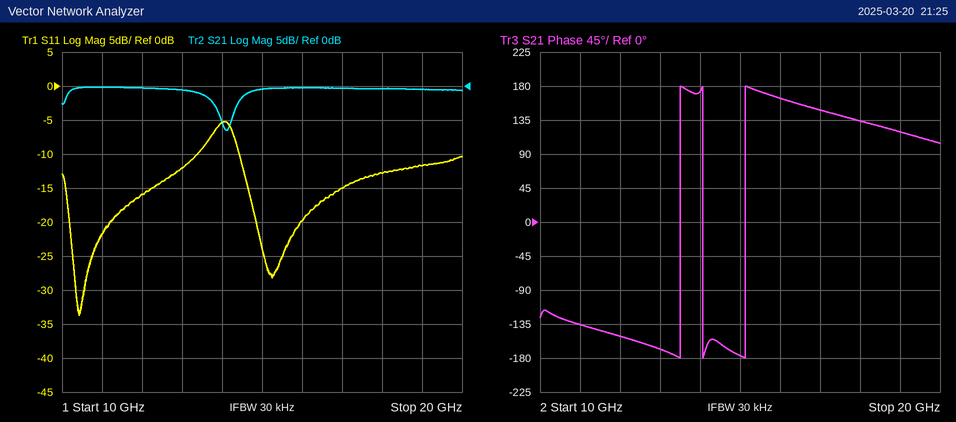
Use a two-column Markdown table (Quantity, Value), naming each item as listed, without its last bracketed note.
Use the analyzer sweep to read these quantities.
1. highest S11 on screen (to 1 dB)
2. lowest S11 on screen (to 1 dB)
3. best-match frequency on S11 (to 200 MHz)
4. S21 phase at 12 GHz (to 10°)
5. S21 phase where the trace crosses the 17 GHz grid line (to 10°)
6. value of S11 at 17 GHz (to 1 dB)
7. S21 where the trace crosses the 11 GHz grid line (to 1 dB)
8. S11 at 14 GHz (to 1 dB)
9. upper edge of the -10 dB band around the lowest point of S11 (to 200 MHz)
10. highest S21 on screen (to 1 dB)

| Quantity | Value |
|---|---|
| highest S11 on screen | -5 dB |
| lowest S11 on screen | -34 dB |
| best-match frequency on S11 | 10.4 GHz |
| S21 phase at 12 GHz | -150° |
| S21 phase where the trace crosses the 17 GHz grid line | 150° |
| value of S11 at 17 GHz | -15 dB |
| S21 where the trace crosses the 11 GHz grid line | 0 dB |
| S11 at 14 GHz | -5 dB |
| upper edge of the -10 dB band around the lowest point of S11 | 13.4 GHz |
| highest S21 on screen | 0 dB |
